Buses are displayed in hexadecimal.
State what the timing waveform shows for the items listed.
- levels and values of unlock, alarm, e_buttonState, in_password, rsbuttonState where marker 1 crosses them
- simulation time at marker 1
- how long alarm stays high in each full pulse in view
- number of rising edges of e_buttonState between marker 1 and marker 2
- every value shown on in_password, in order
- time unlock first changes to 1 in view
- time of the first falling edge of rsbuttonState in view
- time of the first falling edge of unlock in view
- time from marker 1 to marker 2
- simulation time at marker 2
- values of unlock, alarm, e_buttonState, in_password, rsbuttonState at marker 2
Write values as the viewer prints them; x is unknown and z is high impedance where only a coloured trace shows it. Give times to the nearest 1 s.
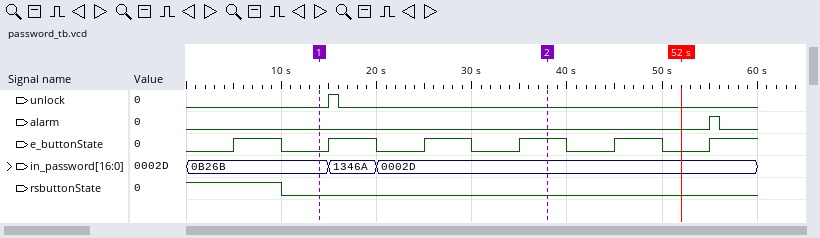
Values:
unlock=0, alarm=0, e_buttonState=0, in_password=0B26B, rsbuttonState=0
14 s
1 s
3
0B26B, 1346A, 0002D
15 s
10 s
16 s
24 s
38 s
unlock=0, alarm=0, e_buttonState=1, in_password=0002D, rsbuttonState=0
